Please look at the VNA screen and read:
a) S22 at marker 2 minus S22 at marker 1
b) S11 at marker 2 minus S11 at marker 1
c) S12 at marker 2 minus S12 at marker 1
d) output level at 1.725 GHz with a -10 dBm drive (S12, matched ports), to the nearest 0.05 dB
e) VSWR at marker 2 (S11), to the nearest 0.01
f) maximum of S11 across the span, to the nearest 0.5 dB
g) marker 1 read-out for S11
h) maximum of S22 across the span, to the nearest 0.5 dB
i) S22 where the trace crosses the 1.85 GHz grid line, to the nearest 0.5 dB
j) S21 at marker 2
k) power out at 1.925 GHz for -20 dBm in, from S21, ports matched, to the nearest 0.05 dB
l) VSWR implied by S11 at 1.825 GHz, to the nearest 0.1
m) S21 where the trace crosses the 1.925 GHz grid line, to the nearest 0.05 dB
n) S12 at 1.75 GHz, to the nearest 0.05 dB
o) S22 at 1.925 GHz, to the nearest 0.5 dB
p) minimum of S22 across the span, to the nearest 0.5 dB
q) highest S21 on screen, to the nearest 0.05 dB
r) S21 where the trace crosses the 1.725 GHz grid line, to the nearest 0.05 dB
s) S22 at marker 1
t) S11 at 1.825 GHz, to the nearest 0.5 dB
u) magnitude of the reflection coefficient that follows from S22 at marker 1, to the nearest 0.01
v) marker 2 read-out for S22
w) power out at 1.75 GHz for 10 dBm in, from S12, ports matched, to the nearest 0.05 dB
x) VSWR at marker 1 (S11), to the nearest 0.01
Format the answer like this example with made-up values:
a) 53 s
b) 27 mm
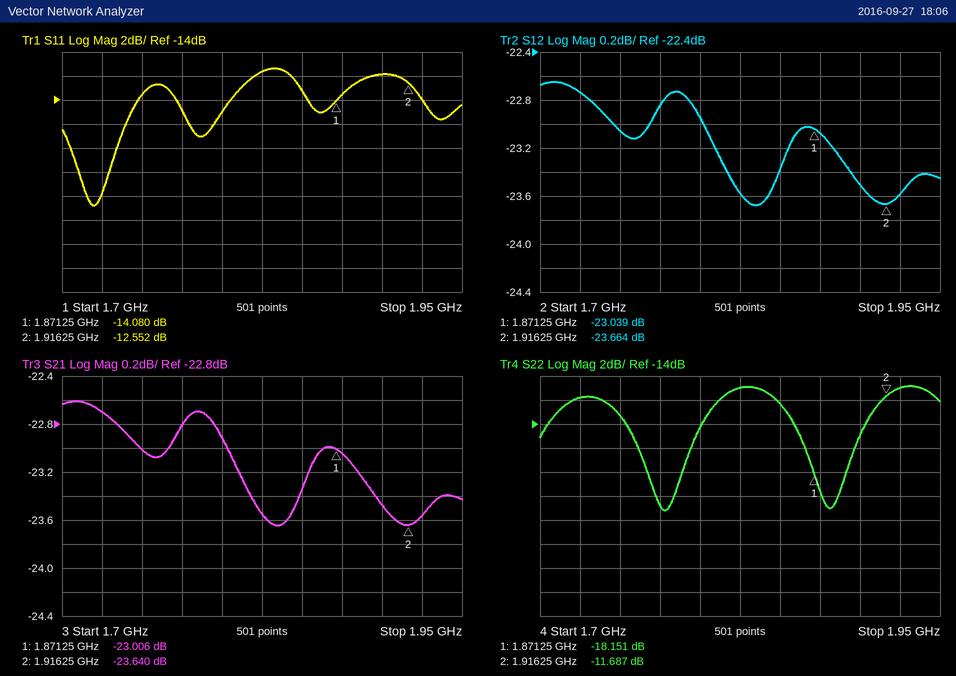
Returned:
a) 6.464 dB
b) 1.528 dB
c) -0.625 dB
d) -32.75 dBm
e) 1.62
f) -11.5 dB
g) -14.080 dB
h) -11.0 dB
i) -12.5 dB
j) -23.640 dB
k) -43.55 dBm
l) 1.7
m) -23.55 dB
n) -23.05 dB
o) -11.0 dB
p) -21.0 dB
q) -22.60 dB
r) -22.70 dB
s) -18.151 dB
t) -11.5 dB
u) 0.12
v) -11.687 dB
w) -13.05 dBm
x) 1.49
